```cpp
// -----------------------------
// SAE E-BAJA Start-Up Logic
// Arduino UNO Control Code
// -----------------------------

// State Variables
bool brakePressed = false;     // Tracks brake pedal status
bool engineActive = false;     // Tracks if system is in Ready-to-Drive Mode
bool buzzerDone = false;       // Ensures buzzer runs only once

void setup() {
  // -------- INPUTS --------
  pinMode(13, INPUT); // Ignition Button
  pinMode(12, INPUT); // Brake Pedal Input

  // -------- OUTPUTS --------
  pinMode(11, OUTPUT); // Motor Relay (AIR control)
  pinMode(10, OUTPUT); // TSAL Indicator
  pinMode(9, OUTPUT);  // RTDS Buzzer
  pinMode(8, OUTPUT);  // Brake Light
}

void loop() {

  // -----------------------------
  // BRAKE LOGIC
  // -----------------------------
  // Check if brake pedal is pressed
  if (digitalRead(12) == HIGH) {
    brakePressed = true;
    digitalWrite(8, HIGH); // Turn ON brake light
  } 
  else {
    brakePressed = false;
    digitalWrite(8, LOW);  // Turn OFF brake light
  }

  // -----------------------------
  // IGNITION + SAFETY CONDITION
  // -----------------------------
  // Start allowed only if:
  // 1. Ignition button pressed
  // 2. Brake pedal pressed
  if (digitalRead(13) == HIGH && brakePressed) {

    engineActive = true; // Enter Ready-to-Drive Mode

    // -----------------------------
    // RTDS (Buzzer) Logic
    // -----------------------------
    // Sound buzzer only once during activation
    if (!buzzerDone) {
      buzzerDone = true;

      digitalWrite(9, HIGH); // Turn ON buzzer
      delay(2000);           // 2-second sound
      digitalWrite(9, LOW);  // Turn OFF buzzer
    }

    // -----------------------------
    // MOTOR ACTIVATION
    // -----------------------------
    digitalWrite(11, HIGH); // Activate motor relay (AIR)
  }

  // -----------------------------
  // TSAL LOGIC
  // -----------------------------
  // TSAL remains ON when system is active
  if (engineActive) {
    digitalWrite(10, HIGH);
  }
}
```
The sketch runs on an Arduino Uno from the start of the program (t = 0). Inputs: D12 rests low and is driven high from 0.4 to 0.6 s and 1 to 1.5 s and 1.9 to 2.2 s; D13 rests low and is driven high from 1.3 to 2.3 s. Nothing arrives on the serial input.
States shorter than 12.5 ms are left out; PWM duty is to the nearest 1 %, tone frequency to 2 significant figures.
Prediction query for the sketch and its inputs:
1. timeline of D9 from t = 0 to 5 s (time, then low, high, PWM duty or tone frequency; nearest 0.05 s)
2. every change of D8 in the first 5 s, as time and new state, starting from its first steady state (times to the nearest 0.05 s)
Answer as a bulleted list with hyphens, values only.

- 0 s low; 1.3 s high; 3.3 s low
- 0 s low; 0.4 s high; 0.6 s low; 1 s high; 3.3 s low
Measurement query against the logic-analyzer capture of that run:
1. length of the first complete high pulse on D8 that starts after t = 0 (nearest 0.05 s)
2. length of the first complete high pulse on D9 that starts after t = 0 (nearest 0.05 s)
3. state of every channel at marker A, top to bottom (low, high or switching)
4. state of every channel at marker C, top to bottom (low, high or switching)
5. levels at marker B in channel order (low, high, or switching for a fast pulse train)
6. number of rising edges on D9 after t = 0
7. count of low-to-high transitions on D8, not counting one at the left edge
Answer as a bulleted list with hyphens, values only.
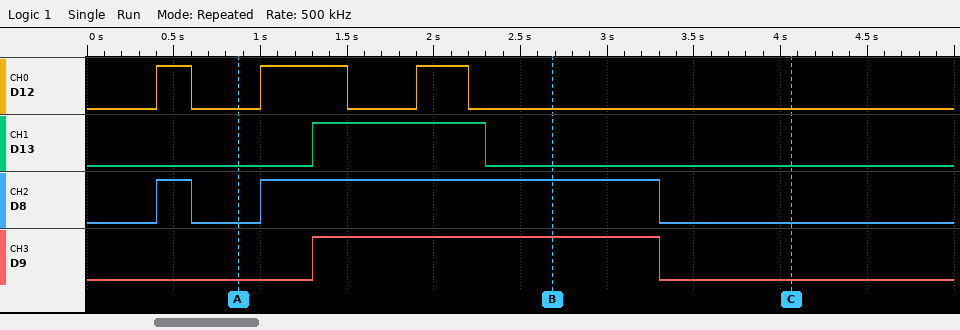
- 0.20 s
- 2.00 s
- D12 low, D13 low, D8 low, D9 low
- D12 low, D13 low, D8 low, D9 low
- D12 low, D13 low, D8 high, D9 high
- 1
- 2
